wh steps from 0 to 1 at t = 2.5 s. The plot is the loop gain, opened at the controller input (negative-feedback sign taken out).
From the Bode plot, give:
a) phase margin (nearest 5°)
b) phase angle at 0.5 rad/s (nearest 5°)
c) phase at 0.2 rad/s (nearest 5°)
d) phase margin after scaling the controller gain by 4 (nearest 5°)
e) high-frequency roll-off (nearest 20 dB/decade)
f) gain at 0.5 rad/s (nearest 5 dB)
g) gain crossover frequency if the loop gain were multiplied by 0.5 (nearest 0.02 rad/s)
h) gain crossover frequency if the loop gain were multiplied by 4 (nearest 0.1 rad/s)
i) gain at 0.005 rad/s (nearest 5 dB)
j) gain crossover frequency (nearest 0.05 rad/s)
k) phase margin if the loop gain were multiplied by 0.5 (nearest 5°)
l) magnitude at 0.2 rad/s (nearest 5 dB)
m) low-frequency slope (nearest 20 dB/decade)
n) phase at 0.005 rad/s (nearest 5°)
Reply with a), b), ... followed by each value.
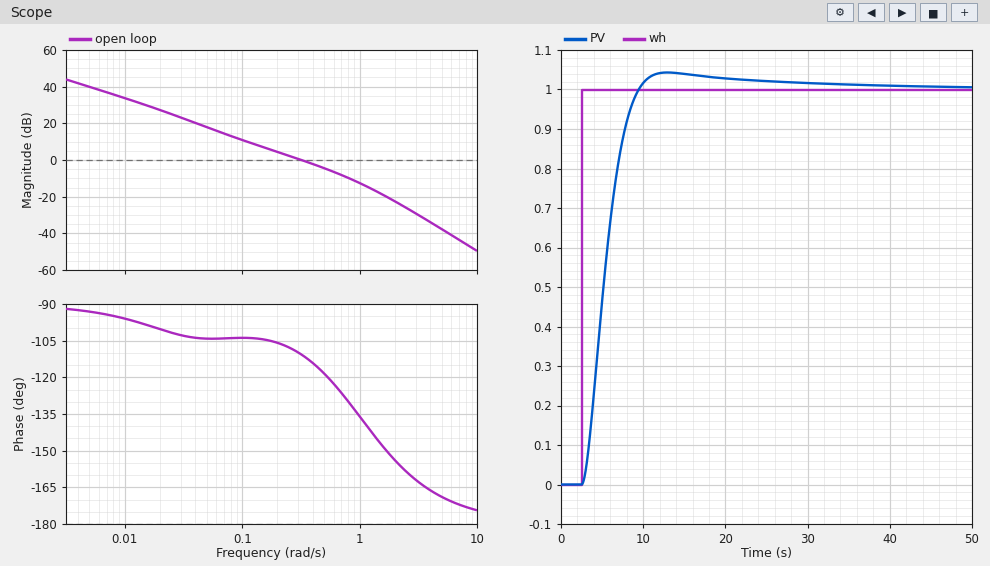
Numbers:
a) 70°
b) -120°
c) -105°
d) 45°
e) -40 dB/decade
f) -5 dB
g) 0.16 rad/s
h) 1.0 rad/s
i) 40 dB
j) 0.30 rad/s
k) 75°
l) 5 dB
m) -20 dB/decade
n) -95°
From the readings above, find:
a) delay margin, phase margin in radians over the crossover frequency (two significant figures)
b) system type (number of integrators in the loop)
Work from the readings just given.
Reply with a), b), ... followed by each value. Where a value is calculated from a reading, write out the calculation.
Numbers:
a) 70 × π / 180 / 0.3 = 4.1 s
b) 1
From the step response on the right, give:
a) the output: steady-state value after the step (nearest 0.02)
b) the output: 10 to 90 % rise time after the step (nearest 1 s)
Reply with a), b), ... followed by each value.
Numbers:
a) 1.00
b) 4 s
